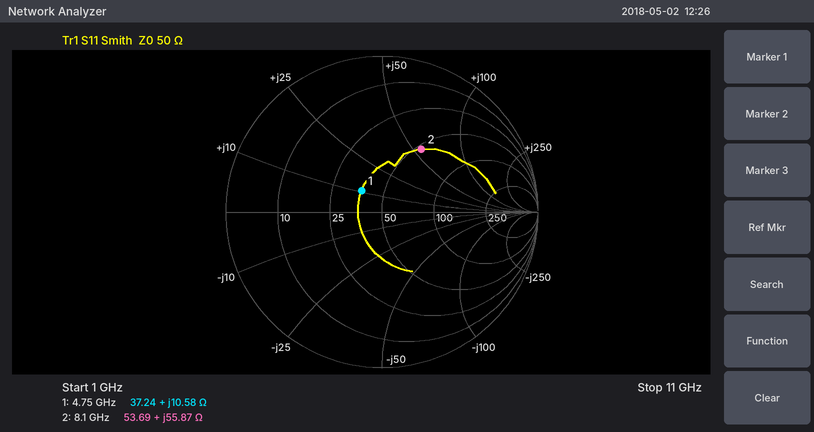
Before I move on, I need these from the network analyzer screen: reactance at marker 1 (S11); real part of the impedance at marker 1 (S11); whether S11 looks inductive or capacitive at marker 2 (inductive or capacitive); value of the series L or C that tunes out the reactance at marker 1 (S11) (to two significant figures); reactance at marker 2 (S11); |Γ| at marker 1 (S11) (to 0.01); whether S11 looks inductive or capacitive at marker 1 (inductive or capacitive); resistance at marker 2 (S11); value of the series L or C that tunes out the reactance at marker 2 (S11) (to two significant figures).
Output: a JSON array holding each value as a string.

["+10.58 Ω", "37.24 Ω", "inductive", "3.2 pF", "+55.87 Ω", "0.19", "inductive", "53.69 Ω", "350 fF"]
